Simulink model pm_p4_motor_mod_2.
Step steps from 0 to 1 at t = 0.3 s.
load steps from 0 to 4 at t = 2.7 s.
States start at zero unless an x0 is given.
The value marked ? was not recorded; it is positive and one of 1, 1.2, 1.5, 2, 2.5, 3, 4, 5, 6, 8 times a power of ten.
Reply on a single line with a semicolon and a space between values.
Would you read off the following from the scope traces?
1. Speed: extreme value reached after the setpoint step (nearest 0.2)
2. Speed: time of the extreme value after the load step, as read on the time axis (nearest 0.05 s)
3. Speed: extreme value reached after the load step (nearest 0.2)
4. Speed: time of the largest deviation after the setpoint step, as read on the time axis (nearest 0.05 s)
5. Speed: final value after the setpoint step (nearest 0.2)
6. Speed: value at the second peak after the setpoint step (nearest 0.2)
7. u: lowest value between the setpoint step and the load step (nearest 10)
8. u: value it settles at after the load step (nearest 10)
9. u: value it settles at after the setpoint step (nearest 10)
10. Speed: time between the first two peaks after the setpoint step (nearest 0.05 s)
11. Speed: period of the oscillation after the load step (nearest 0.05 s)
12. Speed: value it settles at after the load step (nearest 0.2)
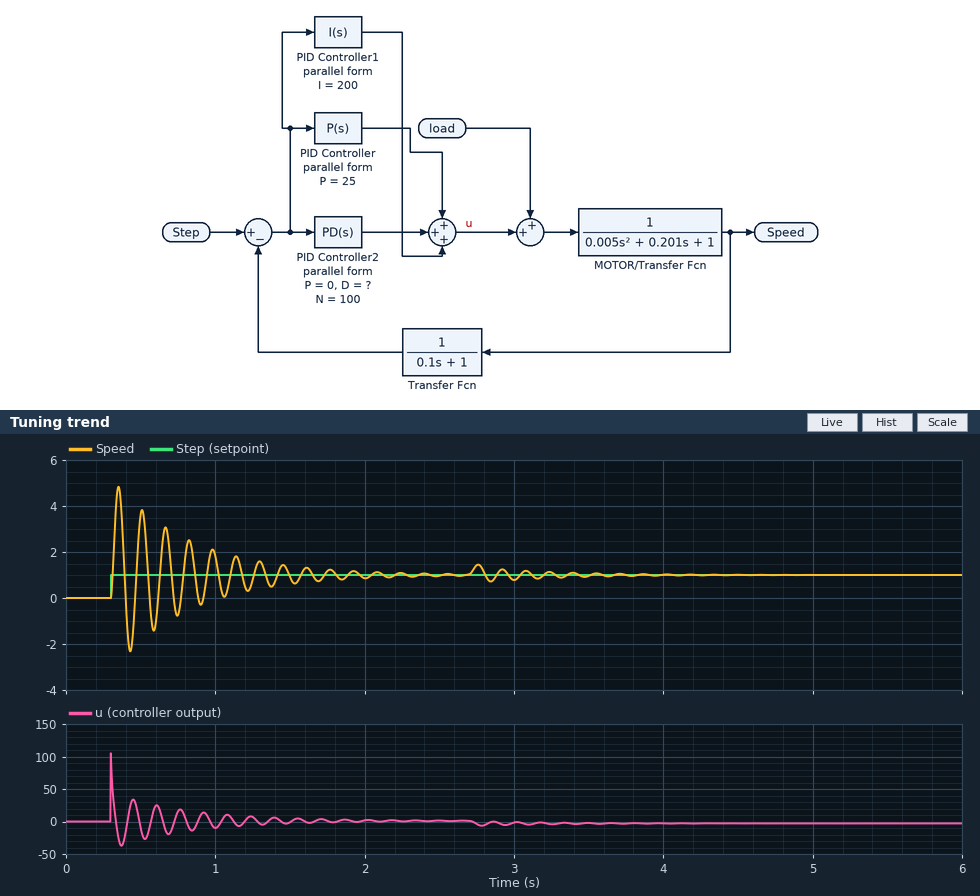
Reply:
4.8; 2.75 s; 1.4; 0.35 s; 1.0; 3.8; -40; 0; 0; 0.15 s; 0.15 s; 1.0
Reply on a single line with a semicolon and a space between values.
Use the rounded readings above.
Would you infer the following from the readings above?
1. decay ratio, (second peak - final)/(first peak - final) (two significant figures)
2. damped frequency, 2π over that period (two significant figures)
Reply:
0.74; 42 rad/s
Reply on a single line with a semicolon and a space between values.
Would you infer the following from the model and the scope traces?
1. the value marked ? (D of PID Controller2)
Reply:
0.8
